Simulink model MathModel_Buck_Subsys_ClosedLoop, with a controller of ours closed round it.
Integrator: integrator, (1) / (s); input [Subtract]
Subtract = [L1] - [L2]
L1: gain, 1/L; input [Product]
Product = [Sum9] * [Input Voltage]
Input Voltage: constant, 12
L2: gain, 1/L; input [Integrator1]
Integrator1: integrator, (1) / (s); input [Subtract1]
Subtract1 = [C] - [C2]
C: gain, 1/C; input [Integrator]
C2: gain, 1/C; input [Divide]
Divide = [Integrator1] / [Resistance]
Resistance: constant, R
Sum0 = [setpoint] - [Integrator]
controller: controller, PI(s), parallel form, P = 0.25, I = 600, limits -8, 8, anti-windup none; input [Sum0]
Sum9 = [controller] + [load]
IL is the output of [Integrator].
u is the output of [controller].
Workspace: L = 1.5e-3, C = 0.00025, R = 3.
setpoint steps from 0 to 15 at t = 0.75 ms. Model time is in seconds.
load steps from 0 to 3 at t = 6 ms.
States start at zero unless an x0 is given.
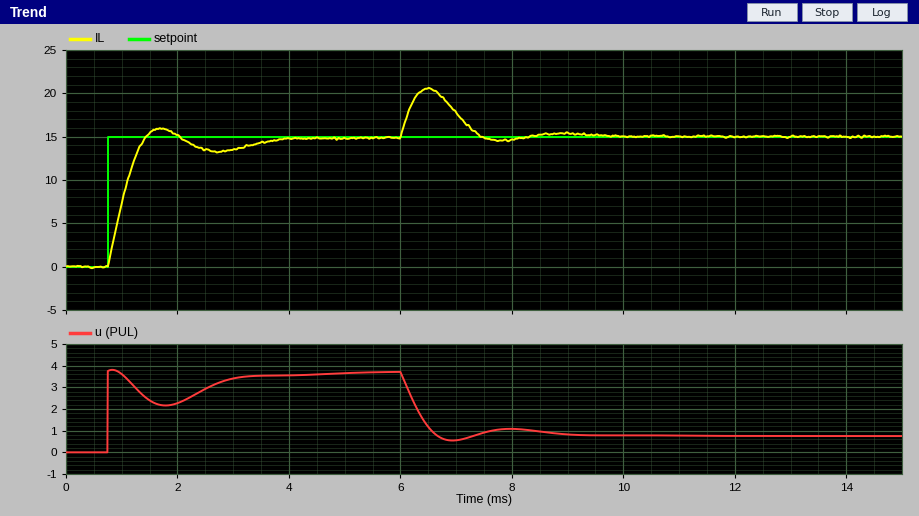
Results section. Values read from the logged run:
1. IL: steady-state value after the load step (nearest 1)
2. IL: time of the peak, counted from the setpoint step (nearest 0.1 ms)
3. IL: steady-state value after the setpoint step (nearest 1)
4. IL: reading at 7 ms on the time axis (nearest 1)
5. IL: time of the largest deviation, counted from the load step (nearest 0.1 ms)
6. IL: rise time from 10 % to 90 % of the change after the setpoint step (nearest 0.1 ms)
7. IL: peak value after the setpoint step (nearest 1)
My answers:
15
0.9 ms
15
18
0.5 ms
0.5 ms
16
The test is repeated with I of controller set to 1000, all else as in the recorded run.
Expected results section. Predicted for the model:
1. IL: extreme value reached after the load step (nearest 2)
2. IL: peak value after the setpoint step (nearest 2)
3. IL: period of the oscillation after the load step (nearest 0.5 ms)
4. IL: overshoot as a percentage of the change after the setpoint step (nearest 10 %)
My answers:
20
18
2.0 ms
20 %
